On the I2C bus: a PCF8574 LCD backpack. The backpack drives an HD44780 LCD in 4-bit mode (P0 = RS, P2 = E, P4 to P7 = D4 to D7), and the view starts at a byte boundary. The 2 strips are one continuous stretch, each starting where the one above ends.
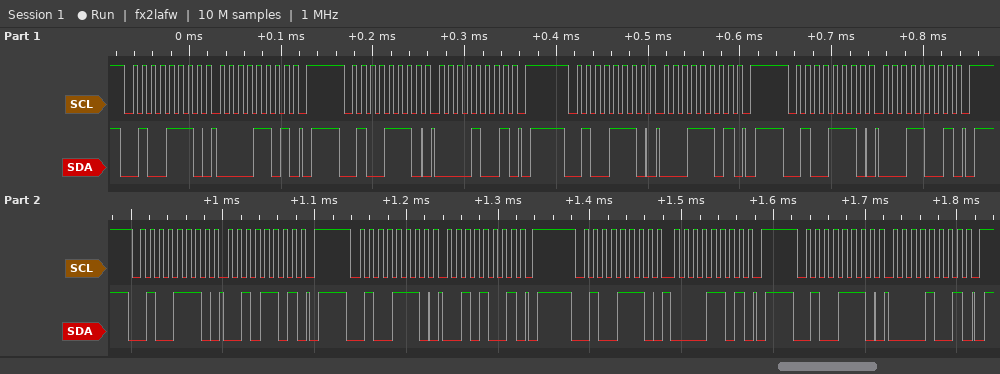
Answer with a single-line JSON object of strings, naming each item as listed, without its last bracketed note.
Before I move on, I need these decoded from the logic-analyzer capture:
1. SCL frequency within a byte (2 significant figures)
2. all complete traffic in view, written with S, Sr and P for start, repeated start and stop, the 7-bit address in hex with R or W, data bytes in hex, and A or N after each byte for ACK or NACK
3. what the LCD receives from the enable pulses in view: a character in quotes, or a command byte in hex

{"SCL frequency within a byte": "100 kHz", "all complete traffic in view, written with S, Sr and P for start, repeated start and stop, the 7-bit address in hex with R or W, data bytes in hex, and A or N after each byte for ACK or NACK": "S 27W A 0D A P S 27W A 09 A P S 27W A 1D A P S 27W A 19 A P S 27W A 2D A P S 27W A 29 A P S 27W A 0D A P S 27W A 09 A P", "what the LCD receives from the enable pulses in view: a character in quotes, or a command byte in hex": "data 0x01 ' '"}
